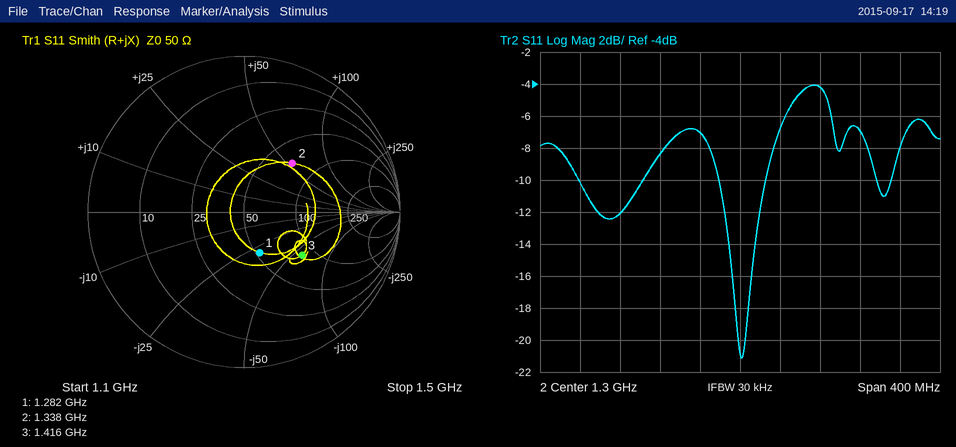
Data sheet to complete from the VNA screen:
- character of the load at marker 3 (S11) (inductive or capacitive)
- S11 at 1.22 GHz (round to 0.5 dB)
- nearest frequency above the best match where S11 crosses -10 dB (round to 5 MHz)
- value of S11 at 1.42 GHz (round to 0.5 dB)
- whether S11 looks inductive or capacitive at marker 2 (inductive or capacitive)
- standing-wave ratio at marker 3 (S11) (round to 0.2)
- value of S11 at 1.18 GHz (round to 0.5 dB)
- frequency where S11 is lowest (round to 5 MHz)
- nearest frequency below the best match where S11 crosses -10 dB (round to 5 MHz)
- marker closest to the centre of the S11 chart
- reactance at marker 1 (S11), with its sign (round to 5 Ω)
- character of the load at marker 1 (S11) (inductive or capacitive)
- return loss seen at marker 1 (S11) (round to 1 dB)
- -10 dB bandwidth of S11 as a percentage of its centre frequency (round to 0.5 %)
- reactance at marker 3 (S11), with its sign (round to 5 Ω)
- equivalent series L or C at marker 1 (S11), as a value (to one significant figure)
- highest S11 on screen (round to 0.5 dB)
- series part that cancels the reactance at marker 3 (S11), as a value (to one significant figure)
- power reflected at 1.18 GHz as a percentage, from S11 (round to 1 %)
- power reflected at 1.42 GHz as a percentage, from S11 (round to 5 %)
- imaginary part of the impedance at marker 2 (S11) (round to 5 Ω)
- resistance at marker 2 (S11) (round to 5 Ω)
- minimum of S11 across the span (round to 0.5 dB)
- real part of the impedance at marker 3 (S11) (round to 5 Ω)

capacitive
-8.5 dB
1.325 GHz
-7.0 dB
inductive
2.8
-12.0 dB
1.300 GHz
1.280 GHz
marker 1
-30 Ω
capacitive
11 dB
3.5 %
-60 Ω
4 pF
-4.0 dB
7 nH
6 %
20 %
+55 Ω
70 Ω
-21.0 dB
85 Ω
